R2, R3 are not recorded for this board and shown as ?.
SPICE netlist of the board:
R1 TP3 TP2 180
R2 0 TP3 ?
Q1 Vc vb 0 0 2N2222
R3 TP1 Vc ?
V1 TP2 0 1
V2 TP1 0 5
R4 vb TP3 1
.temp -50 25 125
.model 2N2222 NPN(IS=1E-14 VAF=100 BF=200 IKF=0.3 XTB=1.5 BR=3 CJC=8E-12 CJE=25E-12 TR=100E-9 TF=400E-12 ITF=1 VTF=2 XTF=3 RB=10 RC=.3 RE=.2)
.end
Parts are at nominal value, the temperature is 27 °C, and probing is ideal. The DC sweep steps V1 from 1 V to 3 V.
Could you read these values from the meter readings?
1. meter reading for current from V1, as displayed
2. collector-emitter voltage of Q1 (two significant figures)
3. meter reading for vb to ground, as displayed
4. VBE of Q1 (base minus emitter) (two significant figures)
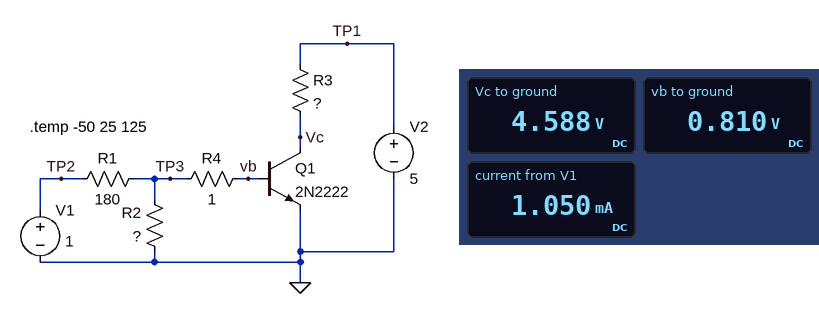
1.050 mA
4.6 V
0.810 V
810 mV
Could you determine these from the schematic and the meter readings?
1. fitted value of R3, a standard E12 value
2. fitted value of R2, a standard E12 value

3.9 Ω
2.2 kΩ
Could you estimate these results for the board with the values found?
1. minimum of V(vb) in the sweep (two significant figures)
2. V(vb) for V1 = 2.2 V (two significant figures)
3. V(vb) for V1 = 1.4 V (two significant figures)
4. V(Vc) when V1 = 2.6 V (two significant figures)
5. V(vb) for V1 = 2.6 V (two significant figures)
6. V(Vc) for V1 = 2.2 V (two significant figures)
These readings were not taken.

810 mV
1.0 V
890 mV
2.8 V
1.0 V
3.1 V
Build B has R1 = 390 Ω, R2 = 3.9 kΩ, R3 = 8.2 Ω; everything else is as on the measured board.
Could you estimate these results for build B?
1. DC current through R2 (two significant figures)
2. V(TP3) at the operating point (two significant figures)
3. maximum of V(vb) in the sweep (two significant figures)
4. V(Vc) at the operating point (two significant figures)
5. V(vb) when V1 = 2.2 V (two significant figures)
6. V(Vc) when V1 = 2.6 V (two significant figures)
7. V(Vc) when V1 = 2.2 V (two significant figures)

200 µA
780 mV
970 mV
4.5 V
910 mV
2.0 V
2.5 V
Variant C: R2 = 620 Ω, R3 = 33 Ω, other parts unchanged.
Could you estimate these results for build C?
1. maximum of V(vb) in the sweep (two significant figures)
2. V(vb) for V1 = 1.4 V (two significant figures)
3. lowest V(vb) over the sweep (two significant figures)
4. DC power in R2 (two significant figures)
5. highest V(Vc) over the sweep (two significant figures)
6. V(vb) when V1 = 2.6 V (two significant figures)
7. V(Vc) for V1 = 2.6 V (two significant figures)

930 mV
840 mV
750 mV
910 µW
4.0 V
910 mV
140 mV
